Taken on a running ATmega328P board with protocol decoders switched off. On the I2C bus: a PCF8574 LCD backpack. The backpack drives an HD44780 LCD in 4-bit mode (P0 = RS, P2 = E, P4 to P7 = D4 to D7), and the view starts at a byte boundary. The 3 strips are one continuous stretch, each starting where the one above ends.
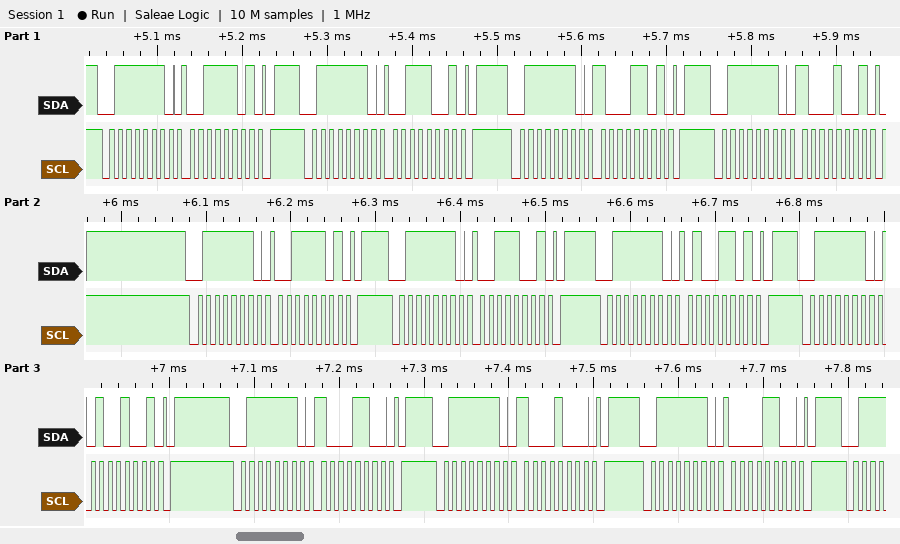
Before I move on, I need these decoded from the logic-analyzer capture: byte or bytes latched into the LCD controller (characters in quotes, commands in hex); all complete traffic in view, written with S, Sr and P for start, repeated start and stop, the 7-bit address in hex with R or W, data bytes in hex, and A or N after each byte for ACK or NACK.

'8' '4'
S 3FW A 3D A P S 3FW A 39 A P S 3FW A 8D A P S 3FW A 89 A P S 3FW A 3D A P S 3FW A 39 A P S 3FW A 4D A P S 3FW A 49 A P S 3FW A 8C A P S 3FW A 88 A P S 3FW A 0C A P
